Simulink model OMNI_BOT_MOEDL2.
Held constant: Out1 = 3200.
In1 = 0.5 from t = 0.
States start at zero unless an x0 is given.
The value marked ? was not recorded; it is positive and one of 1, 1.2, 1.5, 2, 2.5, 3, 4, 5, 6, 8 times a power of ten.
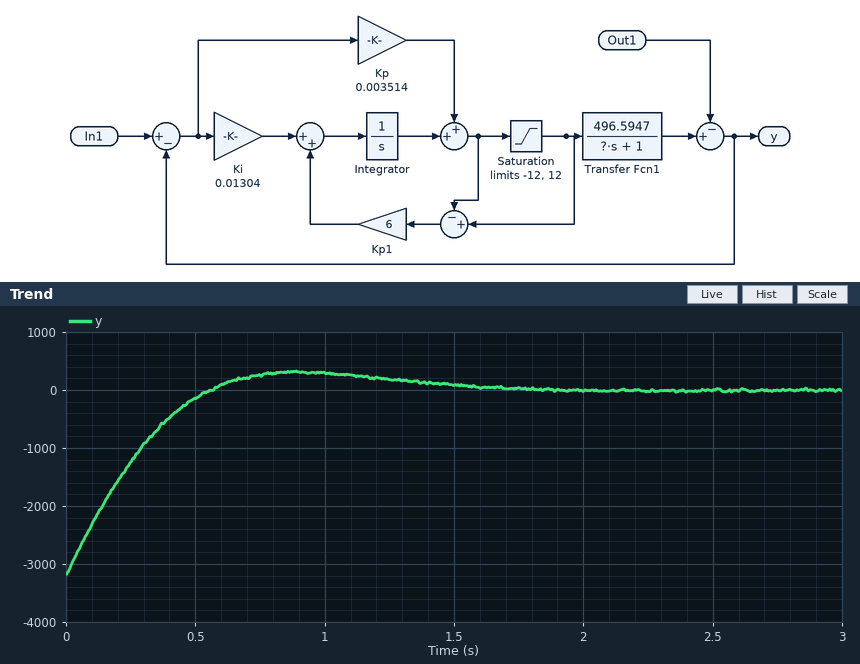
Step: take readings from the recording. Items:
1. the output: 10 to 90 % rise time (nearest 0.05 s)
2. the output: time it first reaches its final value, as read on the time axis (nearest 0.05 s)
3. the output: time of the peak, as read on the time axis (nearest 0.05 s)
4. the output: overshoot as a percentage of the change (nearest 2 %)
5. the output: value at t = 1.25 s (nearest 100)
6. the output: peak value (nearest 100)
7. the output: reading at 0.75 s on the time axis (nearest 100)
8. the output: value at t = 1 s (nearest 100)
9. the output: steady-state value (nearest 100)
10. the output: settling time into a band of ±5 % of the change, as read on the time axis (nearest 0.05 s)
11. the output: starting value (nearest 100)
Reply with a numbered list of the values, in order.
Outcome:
1. 0.40 s
2. 0.55 s
3. 0.90 s
4. 10 %
5. 200
6. 300
7. 300
8. 300
9. 0
10. 1.30 s
11. -3200
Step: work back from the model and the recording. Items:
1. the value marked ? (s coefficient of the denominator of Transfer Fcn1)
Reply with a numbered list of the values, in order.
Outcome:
1. 0.6
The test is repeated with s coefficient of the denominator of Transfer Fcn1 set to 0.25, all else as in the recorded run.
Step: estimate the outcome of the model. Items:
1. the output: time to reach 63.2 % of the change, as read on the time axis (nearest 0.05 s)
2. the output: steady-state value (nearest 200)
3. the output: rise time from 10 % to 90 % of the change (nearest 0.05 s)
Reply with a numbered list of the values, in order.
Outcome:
1. 0.15 s
2. 0
3. 0.35 s
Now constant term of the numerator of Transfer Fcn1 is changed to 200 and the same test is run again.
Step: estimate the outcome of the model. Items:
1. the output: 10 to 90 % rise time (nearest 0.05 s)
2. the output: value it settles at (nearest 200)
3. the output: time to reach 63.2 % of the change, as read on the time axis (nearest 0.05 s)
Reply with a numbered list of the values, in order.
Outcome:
1. 1.30 s
2. -800
3. 0.60 s
